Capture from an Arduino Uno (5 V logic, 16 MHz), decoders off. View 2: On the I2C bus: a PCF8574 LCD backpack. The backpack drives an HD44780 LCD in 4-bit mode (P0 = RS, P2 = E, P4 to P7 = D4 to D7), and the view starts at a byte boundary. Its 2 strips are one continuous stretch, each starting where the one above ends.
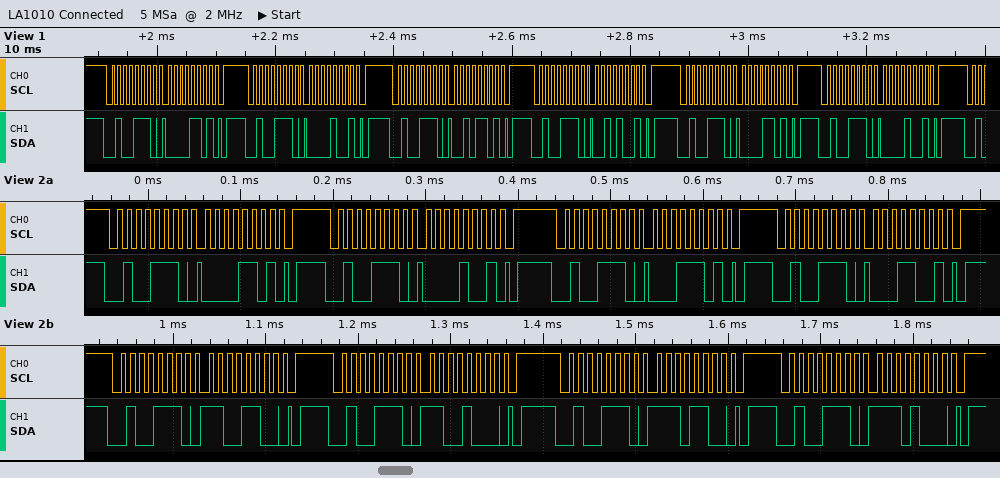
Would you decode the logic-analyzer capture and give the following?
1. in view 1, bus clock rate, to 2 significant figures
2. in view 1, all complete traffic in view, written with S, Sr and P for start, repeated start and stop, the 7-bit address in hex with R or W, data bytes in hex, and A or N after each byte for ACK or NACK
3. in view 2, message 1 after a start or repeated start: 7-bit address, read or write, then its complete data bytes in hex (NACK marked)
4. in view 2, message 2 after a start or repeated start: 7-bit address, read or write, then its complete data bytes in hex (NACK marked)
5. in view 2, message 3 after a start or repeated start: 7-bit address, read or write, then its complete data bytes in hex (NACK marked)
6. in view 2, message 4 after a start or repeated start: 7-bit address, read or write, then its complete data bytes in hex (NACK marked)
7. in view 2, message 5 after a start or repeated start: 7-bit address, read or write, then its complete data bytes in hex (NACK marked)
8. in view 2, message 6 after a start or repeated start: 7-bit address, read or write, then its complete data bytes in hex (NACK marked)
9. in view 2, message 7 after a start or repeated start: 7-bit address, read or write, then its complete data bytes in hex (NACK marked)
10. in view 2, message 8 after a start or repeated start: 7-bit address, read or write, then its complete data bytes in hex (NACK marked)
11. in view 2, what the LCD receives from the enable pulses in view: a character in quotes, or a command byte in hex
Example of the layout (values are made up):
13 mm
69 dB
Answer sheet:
100 kHz
S 27W A 0D A P S 27W A 09 A P S 27W A 2D A P S 27W A 29 A P S 27W A 0D A P S 27W A 09 A P
0x27 write: 0D
0x27 write: 09
0x27 write: 1D
0x27 write: 19
0x27 write: CC
0x27 write: C8
0x27 write: EC
0x27 write: E8
data 0x01 0xCE
